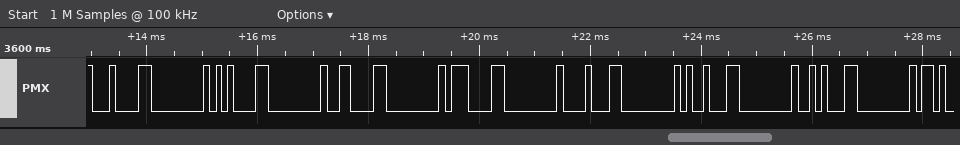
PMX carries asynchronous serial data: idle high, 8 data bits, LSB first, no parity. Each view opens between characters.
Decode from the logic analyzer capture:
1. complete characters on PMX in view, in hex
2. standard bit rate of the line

84, 00, 85, 00, 86, 00, 87, 00, 88, 00, 89, 00, 8A, 00
9600 baud
